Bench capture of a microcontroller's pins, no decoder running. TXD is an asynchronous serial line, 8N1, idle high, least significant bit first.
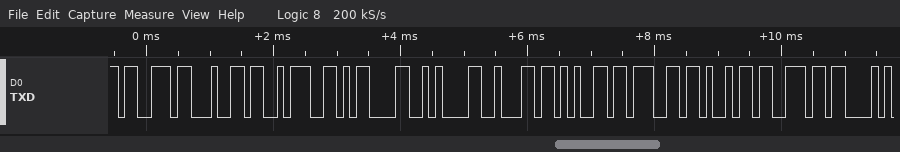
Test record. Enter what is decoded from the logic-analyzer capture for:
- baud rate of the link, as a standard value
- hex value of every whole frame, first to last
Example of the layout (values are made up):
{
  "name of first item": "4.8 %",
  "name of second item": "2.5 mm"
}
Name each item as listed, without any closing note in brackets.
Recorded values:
{
  "baud rate of the link, as a standard value": "9600 baud",
  "hex value of every whole frame, first to last": "0x73 0x64 0x3A 0x0D 0x0A 0x62 0x65 0x67 0x69 0x6E"
}
